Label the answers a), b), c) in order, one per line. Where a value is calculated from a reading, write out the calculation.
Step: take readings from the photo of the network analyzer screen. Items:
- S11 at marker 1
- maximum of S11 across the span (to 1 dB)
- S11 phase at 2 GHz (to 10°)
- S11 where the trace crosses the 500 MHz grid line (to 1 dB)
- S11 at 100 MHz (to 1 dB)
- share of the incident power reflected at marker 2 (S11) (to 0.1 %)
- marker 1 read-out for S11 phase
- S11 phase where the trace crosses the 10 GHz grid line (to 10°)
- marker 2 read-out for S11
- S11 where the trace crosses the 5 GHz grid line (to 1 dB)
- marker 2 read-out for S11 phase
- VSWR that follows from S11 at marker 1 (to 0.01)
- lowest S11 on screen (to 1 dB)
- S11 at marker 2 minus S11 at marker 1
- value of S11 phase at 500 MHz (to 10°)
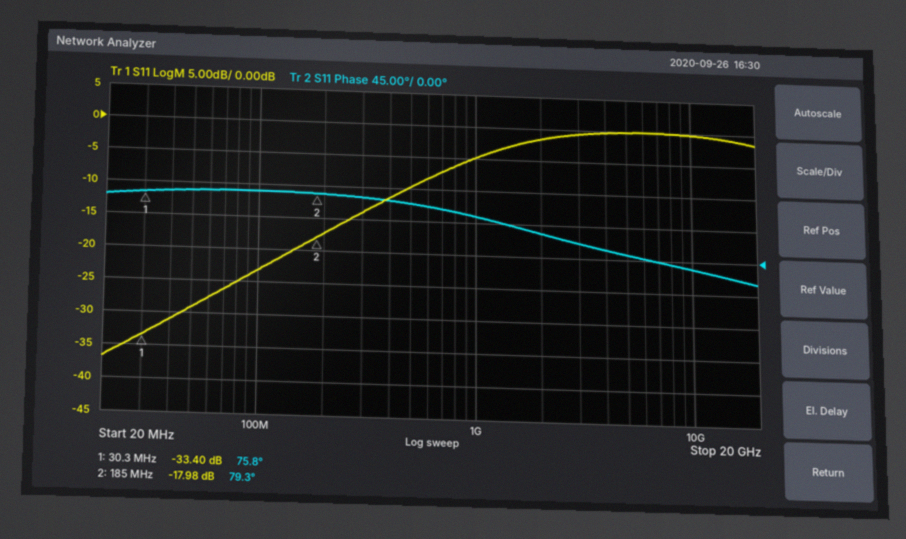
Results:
a) -33.40 dB
b) 0 dB
c) 30°
d) -10 dB
e) -23 dB
f) 10^(-17.98/10) ≈ 1.6 %
g) 75.8°
h) -10°
i) -17.98 dB
j) 0 dB
k) 79.3°
l) (1 + 0.0214)/(1 − 0.0214) ≈ 1.04
m) -37 dB
n) -17.98 − (-33.4) = 15.42 dB
o) 70°
